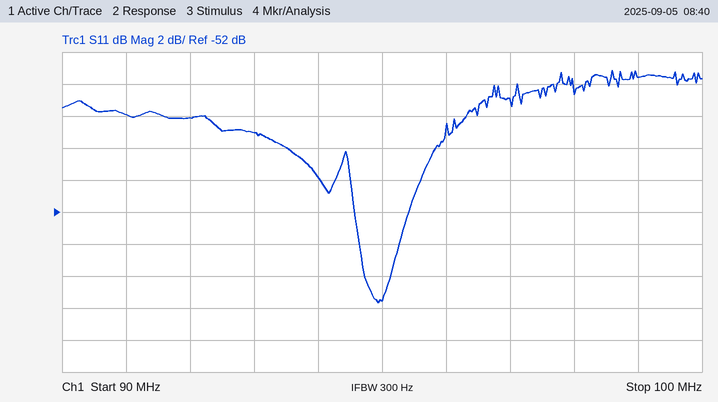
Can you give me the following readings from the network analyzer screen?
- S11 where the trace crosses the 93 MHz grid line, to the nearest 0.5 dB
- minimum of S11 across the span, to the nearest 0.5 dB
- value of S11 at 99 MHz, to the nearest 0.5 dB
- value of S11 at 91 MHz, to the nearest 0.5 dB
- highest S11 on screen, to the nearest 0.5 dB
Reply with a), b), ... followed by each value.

a) -47.0 dB
b) -57.5 dB
c) -43.5 dB
d) -46.0 dB
e) -43.0 dB
